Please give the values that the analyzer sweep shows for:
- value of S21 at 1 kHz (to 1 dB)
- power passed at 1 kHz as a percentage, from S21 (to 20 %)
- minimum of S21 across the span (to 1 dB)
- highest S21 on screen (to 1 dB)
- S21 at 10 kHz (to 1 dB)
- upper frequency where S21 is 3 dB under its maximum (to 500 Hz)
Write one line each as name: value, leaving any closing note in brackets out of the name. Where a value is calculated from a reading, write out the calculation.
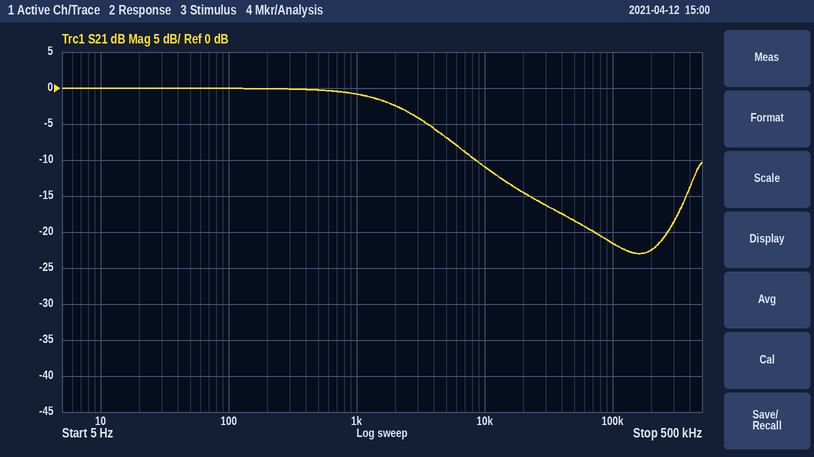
value of S21 at 1 kHz: -1 dB
power passed at 1 kHz as a percentage, from S21: 10^(-1/10) ≈ 79.4 %, so 80 % to the nearest 20 %
minimum of S21 across the span: -23 dB
highest S21 on screen: 0 dB
S21 at 10 kHz: -11 dB
upper frequency where S21 is 3 dB under its maximum: 2.5 kHz
